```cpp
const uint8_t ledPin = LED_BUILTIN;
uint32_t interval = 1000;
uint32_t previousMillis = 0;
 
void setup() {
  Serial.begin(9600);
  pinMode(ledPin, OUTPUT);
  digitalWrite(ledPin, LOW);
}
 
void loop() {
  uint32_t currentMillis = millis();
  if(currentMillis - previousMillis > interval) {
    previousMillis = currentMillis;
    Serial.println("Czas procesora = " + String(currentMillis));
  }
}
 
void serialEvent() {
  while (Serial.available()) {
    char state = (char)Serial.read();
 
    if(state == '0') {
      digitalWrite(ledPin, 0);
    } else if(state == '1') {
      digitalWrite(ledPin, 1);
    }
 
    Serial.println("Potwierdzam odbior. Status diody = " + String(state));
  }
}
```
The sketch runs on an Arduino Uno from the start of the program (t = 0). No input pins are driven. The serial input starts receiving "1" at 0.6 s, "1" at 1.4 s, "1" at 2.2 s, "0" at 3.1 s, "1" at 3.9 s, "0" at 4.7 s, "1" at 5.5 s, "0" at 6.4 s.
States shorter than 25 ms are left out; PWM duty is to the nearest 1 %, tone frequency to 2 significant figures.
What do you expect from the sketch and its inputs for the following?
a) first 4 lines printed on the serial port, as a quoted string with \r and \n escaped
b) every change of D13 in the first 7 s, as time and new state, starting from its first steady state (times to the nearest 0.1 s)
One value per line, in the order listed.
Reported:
"Potwierdzam odbior. Status diody = 1\r\nCzas procesora = 1001\r\nPotwierdzam odbior. Status diody = 1\r\nCzas procesora = 2002\r\n"
0 s low; 0.6 s high; 3.1 s low; 3.9 s high; 4.7 s low; 5.5 s high; 6.4 s low
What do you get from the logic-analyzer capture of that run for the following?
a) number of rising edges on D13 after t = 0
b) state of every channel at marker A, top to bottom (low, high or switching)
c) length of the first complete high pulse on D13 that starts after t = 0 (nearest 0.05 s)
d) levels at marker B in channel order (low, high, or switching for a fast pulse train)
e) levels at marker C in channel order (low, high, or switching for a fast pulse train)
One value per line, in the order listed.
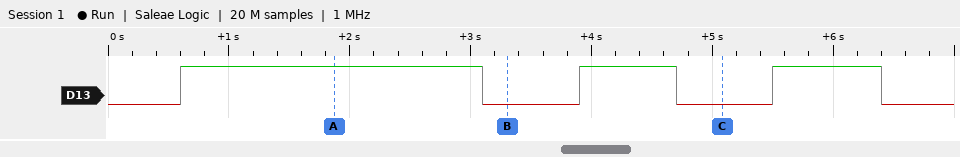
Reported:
3
D13 high
2.50 s
D13 low
D13 low
